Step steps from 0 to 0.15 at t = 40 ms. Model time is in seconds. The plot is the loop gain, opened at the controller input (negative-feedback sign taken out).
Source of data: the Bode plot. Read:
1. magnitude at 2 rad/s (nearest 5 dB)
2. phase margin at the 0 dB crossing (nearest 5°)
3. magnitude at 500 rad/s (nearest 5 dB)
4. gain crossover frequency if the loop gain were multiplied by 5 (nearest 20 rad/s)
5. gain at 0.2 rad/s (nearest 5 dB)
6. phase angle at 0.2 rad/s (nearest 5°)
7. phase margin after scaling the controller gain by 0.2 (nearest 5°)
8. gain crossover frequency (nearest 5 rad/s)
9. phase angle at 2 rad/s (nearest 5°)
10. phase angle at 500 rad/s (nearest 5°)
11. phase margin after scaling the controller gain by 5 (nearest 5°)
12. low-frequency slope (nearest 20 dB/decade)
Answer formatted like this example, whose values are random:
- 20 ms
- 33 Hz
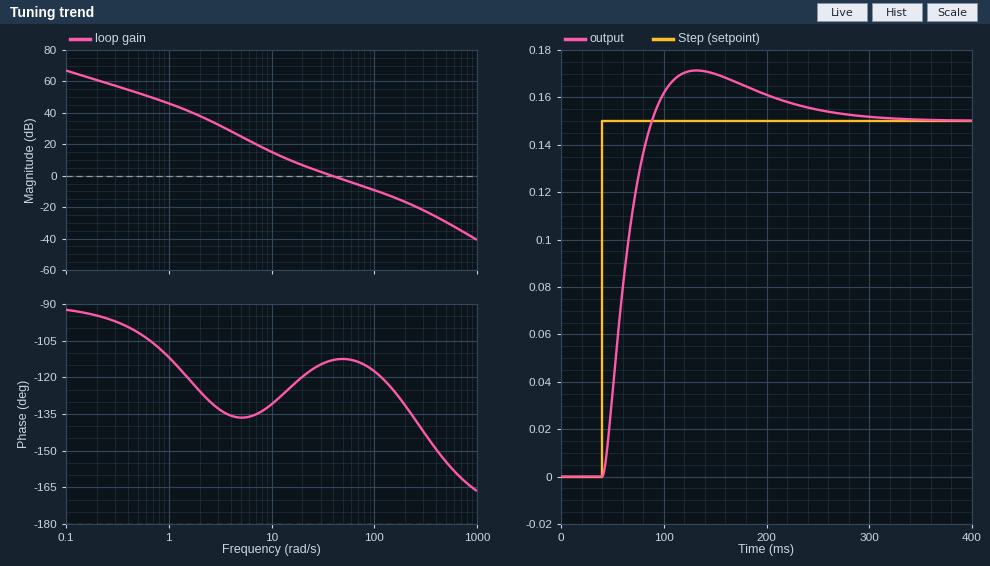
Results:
- 40 dB
- 65°
- -30 dB
- 160 rad/s
- 60 dB
- -95°
- 50°
- 40 rad/s
- -125°
- -155°
- 55°
- -20 dB/decade
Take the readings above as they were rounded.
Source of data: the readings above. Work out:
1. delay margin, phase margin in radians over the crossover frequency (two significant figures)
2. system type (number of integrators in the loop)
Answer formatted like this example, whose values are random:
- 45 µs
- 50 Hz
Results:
- 0.028 s
- 1
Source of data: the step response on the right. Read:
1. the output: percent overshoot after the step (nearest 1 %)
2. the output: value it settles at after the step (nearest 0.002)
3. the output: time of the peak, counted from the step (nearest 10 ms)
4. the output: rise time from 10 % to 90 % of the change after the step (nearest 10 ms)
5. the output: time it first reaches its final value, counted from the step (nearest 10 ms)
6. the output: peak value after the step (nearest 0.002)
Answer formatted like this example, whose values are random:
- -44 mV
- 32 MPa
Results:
- 14 %
- 0.150
- 90 ms
- 30 ms
- 50 ms
- 0.172
